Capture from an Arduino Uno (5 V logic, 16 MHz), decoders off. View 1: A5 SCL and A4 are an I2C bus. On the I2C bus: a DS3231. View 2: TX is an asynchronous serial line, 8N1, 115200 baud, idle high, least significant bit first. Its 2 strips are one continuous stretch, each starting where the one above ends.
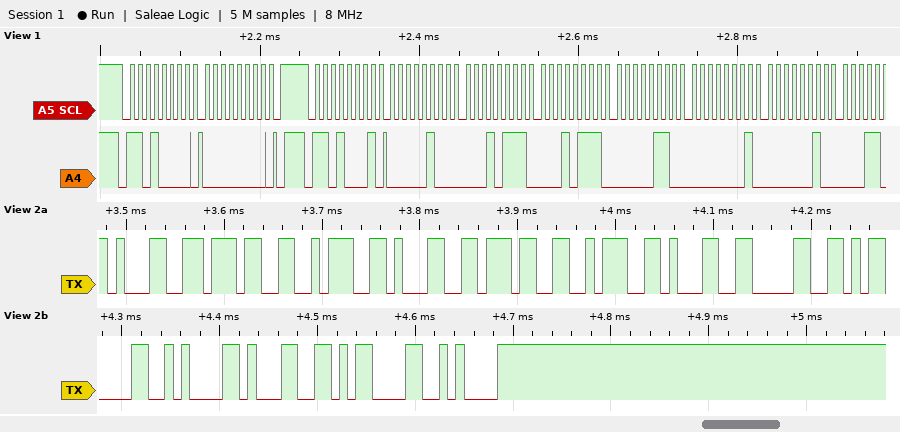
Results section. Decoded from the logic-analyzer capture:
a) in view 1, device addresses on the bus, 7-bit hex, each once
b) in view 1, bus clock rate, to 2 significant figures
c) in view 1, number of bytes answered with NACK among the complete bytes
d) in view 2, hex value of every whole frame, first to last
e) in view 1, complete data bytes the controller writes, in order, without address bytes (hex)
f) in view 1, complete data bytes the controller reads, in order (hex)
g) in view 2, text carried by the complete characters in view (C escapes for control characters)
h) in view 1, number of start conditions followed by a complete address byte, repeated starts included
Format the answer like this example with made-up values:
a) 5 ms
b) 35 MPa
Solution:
a) 0x68
b) 100 kHz
c) 0
d) 31 37 3A 31 37 3A 31 30 0D 0A 31 0D 0A
e) 00
f) 04 17 17 06 01 02
g) "17:17:10\r\n1\r\n"
h) 2
